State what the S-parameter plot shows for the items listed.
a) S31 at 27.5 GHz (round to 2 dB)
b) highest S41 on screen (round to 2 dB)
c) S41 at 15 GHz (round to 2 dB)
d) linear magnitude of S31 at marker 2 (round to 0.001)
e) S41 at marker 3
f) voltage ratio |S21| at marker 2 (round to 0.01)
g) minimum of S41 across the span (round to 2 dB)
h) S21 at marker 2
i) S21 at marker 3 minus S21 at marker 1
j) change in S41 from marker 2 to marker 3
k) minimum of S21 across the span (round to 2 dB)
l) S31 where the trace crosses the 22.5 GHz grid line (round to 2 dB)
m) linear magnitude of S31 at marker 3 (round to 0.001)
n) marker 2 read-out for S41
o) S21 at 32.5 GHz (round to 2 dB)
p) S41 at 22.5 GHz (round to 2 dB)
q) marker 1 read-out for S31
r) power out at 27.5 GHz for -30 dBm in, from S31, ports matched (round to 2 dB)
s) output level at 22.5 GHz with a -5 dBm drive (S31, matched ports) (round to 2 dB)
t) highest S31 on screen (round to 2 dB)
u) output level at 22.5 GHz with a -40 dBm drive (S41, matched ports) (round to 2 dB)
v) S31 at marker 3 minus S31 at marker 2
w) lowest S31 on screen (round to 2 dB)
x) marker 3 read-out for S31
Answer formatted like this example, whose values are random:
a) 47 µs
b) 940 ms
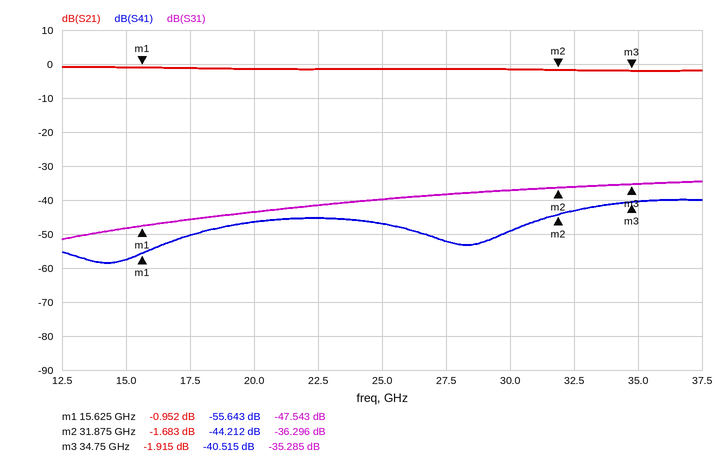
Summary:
a) -38 dB
b) -40 dB
c) -58 dB
d) 0.015
e) -40.515 dB
f) 0.82
g) -58 dB
h) -1.683 dB
i) -0.963 dB
j) 3.697 dB
k) -2 dB
l) -42 dB
m) 0.017
n) -44.212 dB
o) -2 dB
p) -46 dB
q) -47.543 dB
r) -68 dBm
s) -46 dBm
t) -34 dB
u) -86 dBm
v) 1.011 dB
w) -52 dB
x) -35.285 dB
